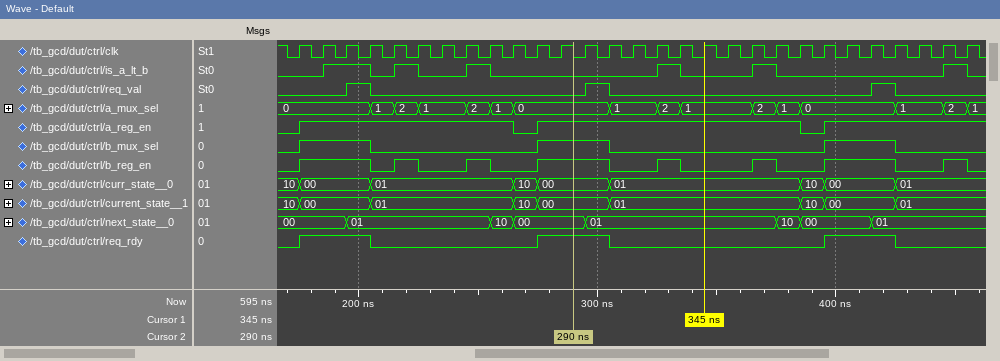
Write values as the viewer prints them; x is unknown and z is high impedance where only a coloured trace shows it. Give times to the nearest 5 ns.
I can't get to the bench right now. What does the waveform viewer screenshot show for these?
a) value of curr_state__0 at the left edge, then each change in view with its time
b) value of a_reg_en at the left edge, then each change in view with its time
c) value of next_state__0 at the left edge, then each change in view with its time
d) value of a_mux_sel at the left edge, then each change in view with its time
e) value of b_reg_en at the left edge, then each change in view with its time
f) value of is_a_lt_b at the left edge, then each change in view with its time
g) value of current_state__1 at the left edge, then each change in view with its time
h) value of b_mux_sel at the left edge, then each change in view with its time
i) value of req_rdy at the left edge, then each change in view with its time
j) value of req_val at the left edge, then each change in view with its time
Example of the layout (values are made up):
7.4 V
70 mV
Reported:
10, 00 at 175 ns, 01 at 205 ns, 10 at 265 ns, 00 at 275 ns, 01 at 305 ns, 10 at 385 ns, 00 at 395 ns, 01 at 425 ns
0, 1 at 175 ns, 0 at 265 ns, 1 at 275 ns, 0 at 385 ns, 1 at 395 ns
00, 01 at 195 ns, 10 at 255 ns, 00 at 265 ns, 01 at 295 ns, 10 at 375 ns, 00 at 385 ns, 01 at 415 ns
0, 1 at 205 ns, 2 at 215 ns, 1 at 225 ns, 2 at 245 ns, 1 at 255 ns, 0 at 265 ns, 1 at 305 ns, 2 at 325 ns, 1 at 335 ns, 2 at 365 ns, 1 at 375 ns, 0 at 385 ns, 1 at 425 ns, 2 at 445 ns, 1 at 455 ns
0, 1 at 175 ns, 0 at 205 ns, 1 at 215 ns, 0 at 225 ns, 1 at 245 ns, 0 at 255 ns, 1 at 275 ns, 0 at 305 ns, 1 at 325 ns, 0 at 335 ns, 1 at 365 ns, 0 at 375 ns, 1 at 395 ns, 0 at 425 ns, 1 at 445 ns, 0 at 455 ns
0, 1 at 185 ns, 0 at 205 ns, 1 at 215 ns, 0 at 225 ns, 1 at 245 ns, 0 at 255 ns, 1 at 325 ns, 0 at 335 ns, 1 at 365 ns, 0 at 375 ns, 1 at 445 ns, 0 at 455 ns
10, 00 at 175 ns, 01 at 205 ns, 10 at 265 ns, 00 at 275 ns, 01 at 305 ns, 10 at 385 ns, 00 at 395 ns, 01 at 425 ns
0, 1 at 175 ns, 0 at 205 ns, 1 at 275 ns, 0 at 305 ns, 1 at 395 ns, 0 at 425 ns
0, 1 at 175 ns, 0 at 205 ns, 1 at 275 ns, 0 at 305 ns, 1 at 395 ns, 0 at 425 ns
0, 1 at 195 ns, 0 at 205 ns, 1 at 295 ns, 0 at 305 ns, 1 at 415 ns, 0 at 425 ns
